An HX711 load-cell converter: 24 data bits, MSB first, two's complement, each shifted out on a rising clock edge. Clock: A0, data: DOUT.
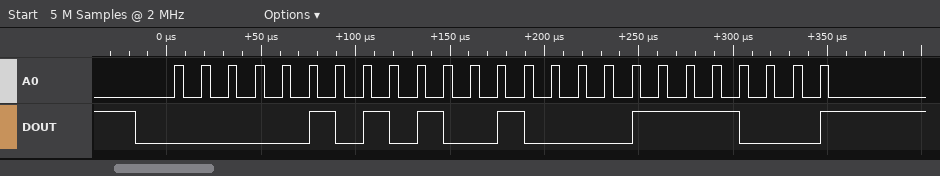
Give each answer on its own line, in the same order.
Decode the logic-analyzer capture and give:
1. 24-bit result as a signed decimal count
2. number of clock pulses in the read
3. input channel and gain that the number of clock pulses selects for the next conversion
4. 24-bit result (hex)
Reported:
346232
25
channel A, gain 128
0x054878
